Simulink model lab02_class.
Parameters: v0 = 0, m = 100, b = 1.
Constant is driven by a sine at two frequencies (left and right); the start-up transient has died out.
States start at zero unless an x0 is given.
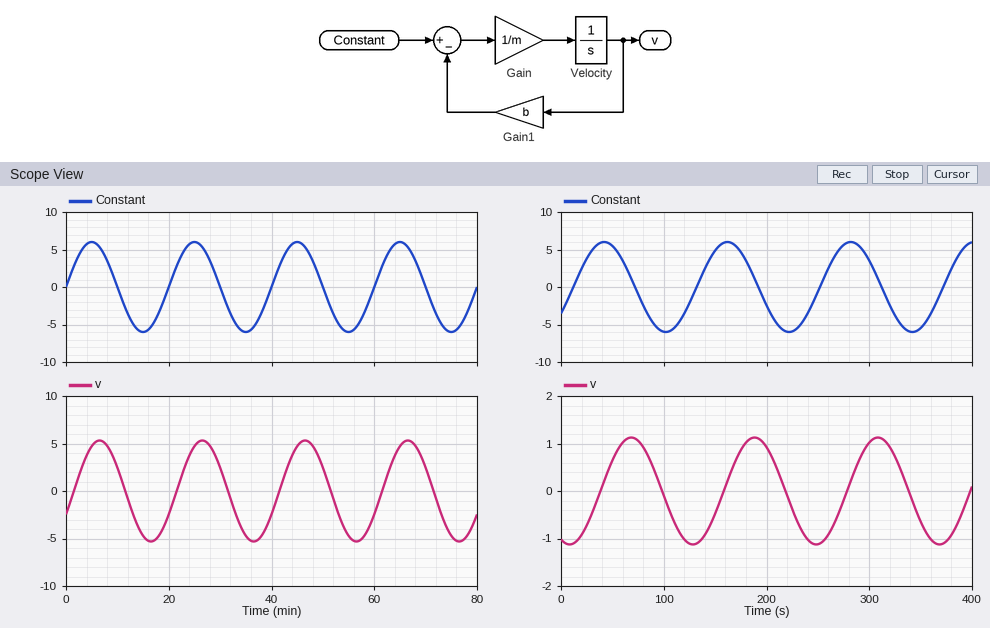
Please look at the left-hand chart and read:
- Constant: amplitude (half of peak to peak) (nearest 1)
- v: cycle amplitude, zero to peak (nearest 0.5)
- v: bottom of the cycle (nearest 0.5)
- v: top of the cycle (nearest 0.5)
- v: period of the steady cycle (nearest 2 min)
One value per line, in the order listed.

6
5.5
-5.5
5.5
20 min
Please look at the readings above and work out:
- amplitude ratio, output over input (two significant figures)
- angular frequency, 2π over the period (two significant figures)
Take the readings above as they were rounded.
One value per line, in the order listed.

0.92
0.31 rad/min
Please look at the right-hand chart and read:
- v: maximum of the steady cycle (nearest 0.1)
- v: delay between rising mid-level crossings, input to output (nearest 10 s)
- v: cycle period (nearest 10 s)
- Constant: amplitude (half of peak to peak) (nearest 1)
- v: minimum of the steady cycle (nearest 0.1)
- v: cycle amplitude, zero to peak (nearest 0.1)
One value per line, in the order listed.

1.1
30 s
120 s
6
-1.1
1.1
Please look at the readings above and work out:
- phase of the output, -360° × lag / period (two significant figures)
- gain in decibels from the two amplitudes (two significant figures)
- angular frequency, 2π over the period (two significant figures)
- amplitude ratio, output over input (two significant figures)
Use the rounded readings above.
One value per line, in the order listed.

-90°
-15 dB
0.052 rad/s
0.18
